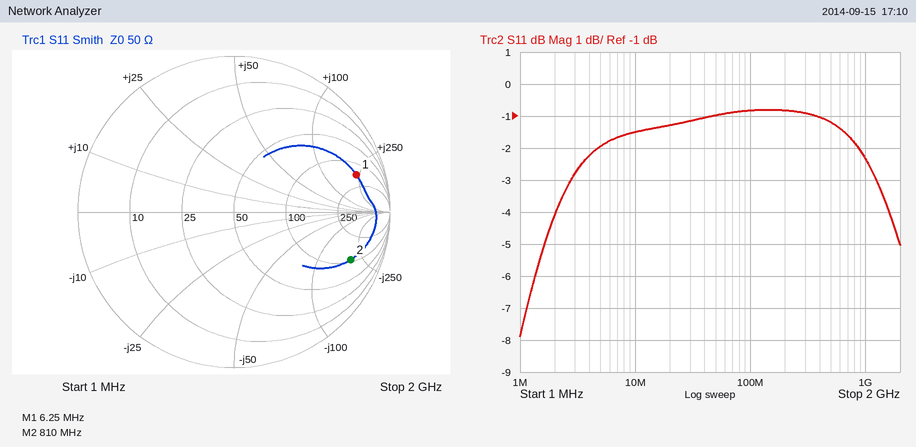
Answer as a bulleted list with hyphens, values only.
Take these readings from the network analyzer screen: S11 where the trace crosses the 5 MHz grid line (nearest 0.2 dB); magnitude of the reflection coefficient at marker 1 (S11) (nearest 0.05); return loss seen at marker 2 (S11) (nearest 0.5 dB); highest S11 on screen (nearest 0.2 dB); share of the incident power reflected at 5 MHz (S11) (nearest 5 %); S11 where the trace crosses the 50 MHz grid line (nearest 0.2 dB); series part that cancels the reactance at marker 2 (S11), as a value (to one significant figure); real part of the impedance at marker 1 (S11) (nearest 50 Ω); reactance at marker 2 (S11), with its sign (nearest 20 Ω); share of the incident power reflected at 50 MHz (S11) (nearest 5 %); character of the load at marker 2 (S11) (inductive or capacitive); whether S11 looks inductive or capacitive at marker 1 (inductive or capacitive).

- -2.0 dB
- 0.80
- 2.0 dB
- -0.8 dB
- 65 %
- -1.0 dB
- 40 nH
- 150 Ω
- -200 Ω
- 80 %
- capacitive
- inductive
